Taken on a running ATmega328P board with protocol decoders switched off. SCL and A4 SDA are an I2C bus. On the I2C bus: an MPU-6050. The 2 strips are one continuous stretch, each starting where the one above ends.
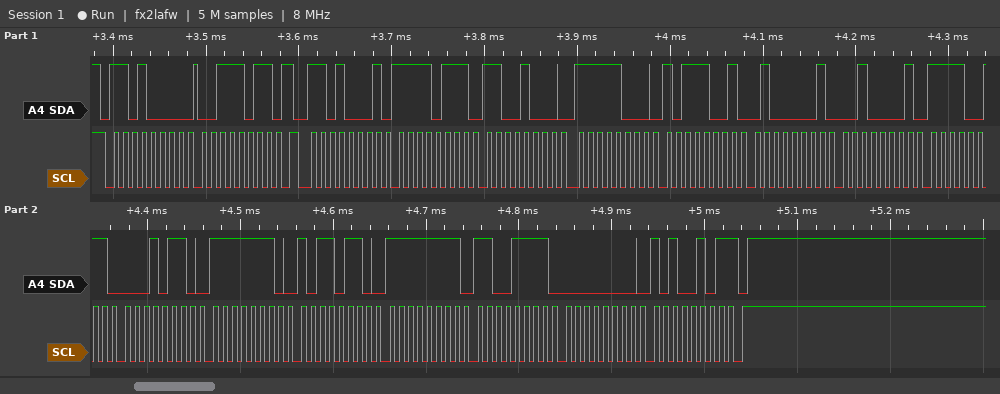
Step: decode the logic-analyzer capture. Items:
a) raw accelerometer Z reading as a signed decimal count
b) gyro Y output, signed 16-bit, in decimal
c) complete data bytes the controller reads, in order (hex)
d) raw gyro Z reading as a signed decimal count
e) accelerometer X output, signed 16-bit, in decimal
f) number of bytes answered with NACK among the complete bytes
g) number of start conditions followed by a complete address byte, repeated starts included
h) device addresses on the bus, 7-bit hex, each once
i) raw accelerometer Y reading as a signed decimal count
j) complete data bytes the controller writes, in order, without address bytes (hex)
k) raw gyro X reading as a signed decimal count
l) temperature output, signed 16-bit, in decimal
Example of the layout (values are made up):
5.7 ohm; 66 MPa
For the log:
16673; -49; F7 C8 F8 B9 41 21 F3 16 FE B6 FF CF 00 A5; 165; -2104; 1; 2; 0x68; -1863; 3B; -330; -3306
